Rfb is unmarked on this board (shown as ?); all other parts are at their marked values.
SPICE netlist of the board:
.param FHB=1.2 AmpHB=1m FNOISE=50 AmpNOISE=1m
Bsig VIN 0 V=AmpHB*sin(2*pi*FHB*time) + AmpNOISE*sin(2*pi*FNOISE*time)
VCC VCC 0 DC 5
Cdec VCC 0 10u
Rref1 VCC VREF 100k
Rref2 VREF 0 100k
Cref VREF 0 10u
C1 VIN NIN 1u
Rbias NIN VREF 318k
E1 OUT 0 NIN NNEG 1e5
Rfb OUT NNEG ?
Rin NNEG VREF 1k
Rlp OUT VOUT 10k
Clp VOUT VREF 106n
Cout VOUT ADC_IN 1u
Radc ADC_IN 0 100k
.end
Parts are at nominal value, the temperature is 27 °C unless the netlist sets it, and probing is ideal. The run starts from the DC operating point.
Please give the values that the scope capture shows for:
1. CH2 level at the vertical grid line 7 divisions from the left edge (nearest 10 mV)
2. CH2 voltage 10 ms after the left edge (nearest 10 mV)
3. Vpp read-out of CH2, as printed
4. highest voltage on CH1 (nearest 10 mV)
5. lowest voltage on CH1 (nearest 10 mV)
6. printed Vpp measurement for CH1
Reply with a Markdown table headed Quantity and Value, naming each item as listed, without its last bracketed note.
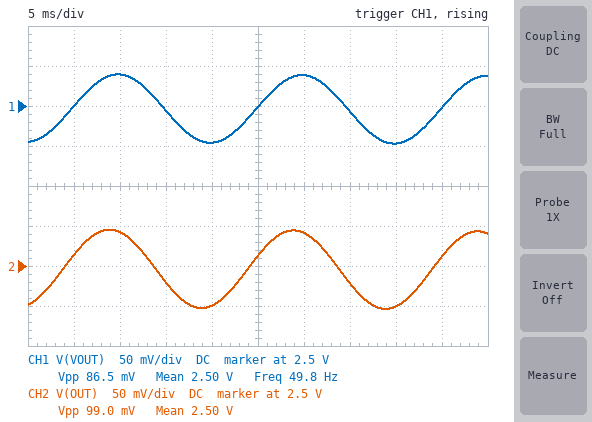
| Quantity | Value |
|---|---|
| CH2 level at the vertical grid line 7 divisions from the left edge | 2.48 V |
| CH2 voltage 10 ms after the left edge | 2.54 V |
| Vpp read-out of CH2, as printed | 99.0 mV |
| highest voltage on CH1 | 2.54 V |
| lowest voltage on CH1 | 2.45 V |
| printed Vpp measurement for CH1 | 86.5 mV |
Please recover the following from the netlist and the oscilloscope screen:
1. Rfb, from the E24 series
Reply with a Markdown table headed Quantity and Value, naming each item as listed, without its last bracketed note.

| Quantity | Value |
|---|---|
| Rfb, from the E24 series | 91 kΩ |
